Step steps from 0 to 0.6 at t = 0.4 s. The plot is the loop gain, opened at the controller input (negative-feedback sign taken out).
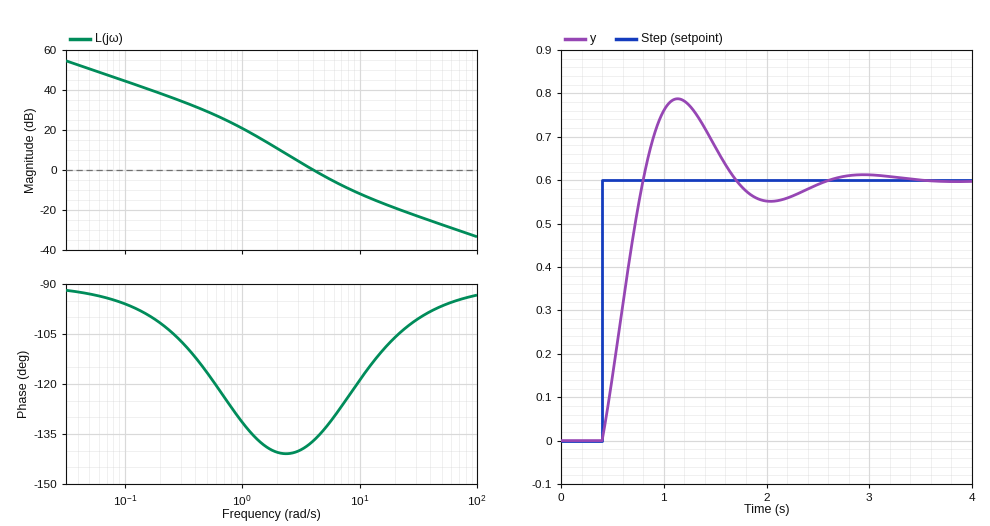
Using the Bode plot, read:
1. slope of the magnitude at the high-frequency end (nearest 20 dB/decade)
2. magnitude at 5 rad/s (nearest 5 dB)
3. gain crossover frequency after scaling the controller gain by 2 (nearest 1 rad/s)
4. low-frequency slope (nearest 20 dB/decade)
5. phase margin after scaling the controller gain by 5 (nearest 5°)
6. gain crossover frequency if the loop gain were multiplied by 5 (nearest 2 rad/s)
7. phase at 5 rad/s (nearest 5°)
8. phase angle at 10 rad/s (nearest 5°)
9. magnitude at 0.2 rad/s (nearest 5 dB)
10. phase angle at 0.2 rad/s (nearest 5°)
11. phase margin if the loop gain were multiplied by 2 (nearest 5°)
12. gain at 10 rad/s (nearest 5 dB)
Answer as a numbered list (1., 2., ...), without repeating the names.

1. -20 dB/decade
2. -5 dB
3. 6 rad/s
4. -20 dB/decade
5. 65°
6. 12 rad/s
7. -135°
8. -120°
9. 40 dB
10. -100°
11. 50°
12. -10 dB
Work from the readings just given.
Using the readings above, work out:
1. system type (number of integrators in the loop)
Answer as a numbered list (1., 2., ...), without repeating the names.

1. 1
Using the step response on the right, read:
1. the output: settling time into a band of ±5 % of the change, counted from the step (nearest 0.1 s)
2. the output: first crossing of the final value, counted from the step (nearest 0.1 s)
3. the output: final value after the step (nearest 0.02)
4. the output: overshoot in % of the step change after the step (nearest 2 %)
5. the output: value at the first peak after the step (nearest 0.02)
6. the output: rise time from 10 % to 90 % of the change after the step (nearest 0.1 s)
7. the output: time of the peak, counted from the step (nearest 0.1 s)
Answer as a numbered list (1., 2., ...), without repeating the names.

1. 1.9 s
2. 0.4 s
3. 0.60
4. 32 %
5. 0.78
6. 0.3 s
7. 0.7 s
